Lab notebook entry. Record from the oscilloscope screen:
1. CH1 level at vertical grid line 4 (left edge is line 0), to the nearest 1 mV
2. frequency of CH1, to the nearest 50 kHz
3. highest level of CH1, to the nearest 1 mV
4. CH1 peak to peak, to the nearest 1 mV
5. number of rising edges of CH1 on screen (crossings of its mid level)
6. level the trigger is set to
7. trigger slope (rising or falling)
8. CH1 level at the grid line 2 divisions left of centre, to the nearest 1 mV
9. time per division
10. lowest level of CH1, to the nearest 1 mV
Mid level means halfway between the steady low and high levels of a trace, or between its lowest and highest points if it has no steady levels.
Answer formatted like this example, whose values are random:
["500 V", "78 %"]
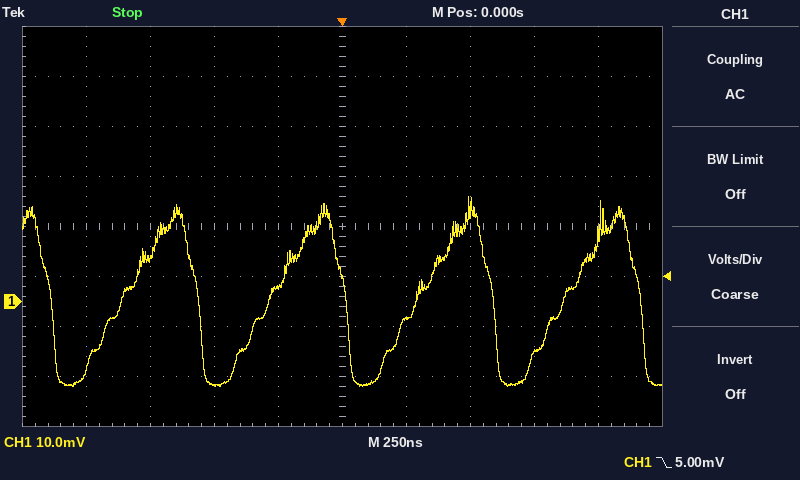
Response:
["3 mV", "1.75 MHz", "21 mV", "38 mV", "4", "5.00 mV", "falling", "-17 mV", "250 ns", "-17 mV"]
